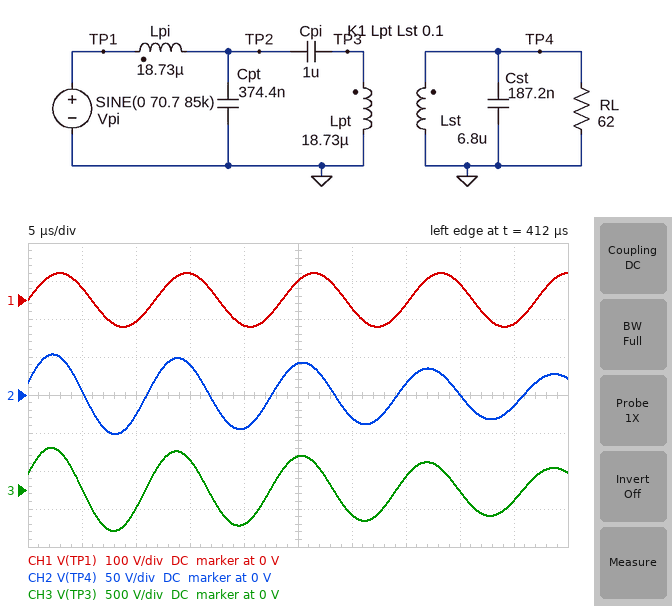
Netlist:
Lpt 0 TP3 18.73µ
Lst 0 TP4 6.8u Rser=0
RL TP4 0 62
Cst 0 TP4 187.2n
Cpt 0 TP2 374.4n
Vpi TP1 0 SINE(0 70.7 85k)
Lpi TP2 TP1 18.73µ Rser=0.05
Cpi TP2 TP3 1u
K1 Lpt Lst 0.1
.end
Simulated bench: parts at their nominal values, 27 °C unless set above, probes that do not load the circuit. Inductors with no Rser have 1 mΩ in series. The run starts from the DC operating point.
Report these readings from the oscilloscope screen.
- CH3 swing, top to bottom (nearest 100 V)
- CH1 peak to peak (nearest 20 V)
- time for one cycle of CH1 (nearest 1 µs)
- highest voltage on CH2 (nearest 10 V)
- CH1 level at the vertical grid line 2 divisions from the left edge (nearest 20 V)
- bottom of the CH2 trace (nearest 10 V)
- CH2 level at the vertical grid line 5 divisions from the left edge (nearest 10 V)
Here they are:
1.1 kV
140 V
12 µs
50 V
-60 V
-50 V
40 V
